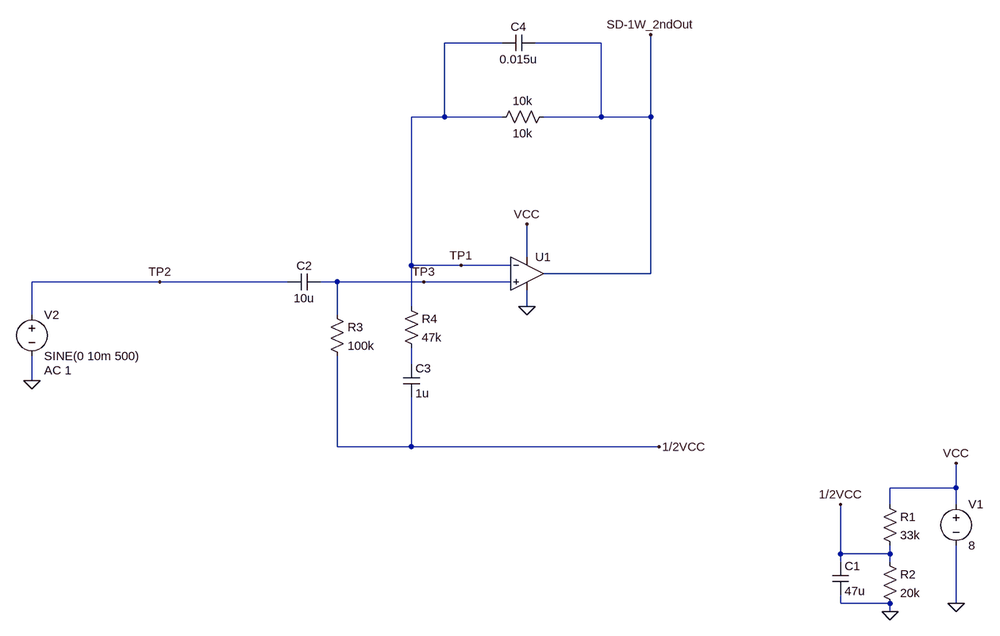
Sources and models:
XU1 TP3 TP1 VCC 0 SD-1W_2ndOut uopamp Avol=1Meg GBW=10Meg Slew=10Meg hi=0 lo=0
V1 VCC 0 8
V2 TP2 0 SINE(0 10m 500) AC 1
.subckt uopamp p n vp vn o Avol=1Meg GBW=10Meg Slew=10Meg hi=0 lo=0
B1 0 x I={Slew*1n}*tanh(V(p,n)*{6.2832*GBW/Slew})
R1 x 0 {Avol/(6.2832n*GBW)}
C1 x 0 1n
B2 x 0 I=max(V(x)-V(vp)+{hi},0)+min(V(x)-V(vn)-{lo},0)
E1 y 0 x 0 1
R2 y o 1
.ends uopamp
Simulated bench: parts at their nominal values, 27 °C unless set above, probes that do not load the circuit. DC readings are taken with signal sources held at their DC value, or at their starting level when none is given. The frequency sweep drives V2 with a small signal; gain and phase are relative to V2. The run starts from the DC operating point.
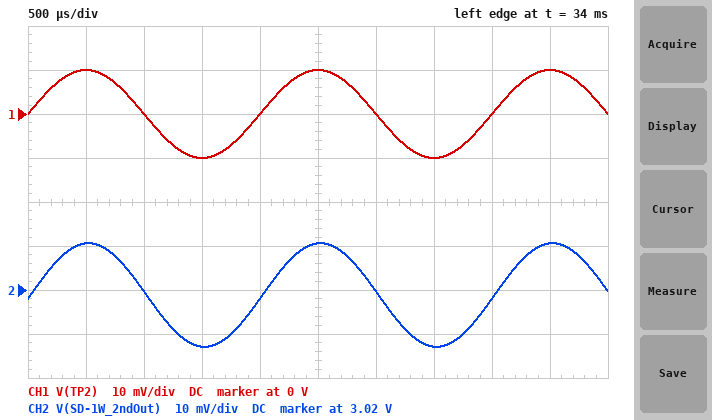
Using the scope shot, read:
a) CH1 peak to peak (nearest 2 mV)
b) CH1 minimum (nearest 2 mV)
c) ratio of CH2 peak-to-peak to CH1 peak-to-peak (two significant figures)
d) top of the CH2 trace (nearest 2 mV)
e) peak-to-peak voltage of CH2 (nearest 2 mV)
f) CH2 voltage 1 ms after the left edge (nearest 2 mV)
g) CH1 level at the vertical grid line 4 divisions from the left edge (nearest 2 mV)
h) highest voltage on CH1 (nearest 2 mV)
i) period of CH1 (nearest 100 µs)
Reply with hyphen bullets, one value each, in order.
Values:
- 20 mV
- -10 mV
- 1.2
- 3.030 V
- 24 mV
- 3.020 V
- 0 V
- 10 mV
- 2.0 ms
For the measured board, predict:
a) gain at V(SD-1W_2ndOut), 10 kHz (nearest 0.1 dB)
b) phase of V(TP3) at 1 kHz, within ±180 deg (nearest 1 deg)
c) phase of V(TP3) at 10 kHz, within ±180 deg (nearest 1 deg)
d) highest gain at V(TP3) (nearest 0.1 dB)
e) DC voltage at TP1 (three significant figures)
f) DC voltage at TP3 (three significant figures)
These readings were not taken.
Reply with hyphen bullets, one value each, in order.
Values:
- 0 dB
- 0 deg
- 0 deg
- 0 dB
- 3.02 V
- 3.02 V
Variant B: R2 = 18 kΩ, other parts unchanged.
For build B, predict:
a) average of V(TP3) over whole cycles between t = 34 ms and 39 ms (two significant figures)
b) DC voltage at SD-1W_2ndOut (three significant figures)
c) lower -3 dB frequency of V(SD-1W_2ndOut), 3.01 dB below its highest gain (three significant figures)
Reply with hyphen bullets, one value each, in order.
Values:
- 2.8 V
- 2.82 V
- 265 mHz
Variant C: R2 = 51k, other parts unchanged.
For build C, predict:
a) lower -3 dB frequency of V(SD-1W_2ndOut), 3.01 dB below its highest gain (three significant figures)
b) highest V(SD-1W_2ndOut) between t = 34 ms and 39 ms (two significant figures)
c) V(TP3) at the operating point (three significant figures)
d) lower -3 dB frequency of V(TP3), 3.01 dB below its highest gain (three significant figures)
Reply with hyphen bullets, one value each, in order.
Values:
- 279 mHz
- 4.9 V
- 4.86 V
- 153 mHz
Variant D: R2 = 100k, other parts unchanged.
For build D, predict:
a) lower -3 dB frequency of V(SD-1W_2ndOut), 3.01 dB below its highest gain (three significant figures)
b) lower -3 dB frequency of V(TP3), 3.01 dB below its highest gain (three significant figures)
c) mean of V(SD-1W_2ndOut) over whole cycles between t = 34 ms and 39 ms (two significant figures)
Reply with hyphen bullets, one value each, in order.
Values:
- 285 mHz
- 156 mHz
- 6.0 V
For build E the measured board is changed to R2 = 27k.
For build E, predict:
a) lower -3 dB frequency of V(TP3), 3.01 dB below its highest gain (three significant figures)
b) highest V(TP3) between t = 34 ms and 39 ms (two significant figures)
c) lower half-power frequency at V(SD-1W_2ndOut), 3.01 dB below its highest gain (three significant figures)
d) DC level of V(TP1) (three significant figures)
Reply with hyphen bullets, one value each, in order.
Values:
- 151 mHz
- 3.6 V
- 271 mHz
- 3.60 V
